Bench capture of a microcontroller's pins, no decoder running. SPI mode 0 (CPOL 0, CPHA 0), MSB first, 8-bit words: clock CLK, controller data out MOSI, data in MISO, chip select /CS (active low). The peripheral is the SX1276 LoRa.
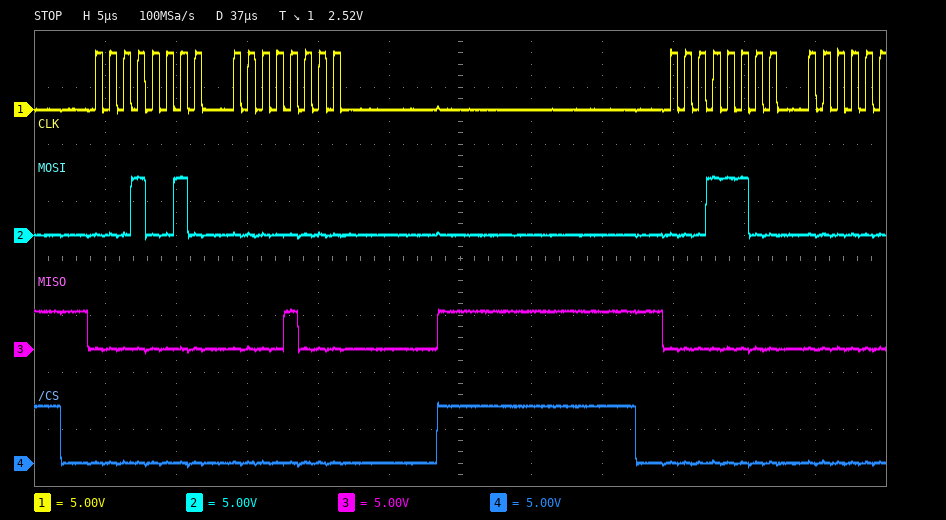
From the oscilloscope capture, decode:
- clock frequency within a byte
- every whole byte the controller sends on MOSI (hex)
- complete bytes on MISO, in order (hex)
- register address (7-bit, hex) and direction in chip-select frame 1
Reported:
1 MHz
12 00 1C
00 08 00
0x12 read
